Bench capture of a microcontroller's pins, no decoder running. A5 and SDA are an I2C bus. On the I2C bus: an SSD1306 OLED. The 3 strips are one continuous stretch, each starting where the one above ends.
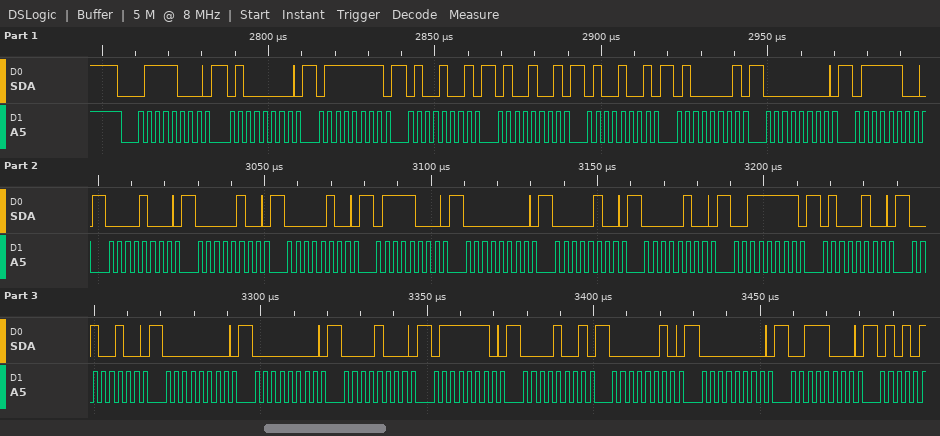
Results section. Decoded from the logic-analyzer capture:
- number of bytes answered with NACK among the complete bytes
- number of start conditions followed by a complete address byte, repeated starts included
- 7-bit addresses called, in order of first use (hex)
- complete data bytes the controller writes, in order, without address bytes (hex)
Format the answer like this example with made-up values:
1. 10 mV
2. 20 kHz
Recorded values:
1. 0
2. 1
3. 0x3C
4. 40 7F 49 49 49 41 00 7C 08 04 04 78 00 04 04 3F 44 24 00 00 08 7E 09 02 00 38
